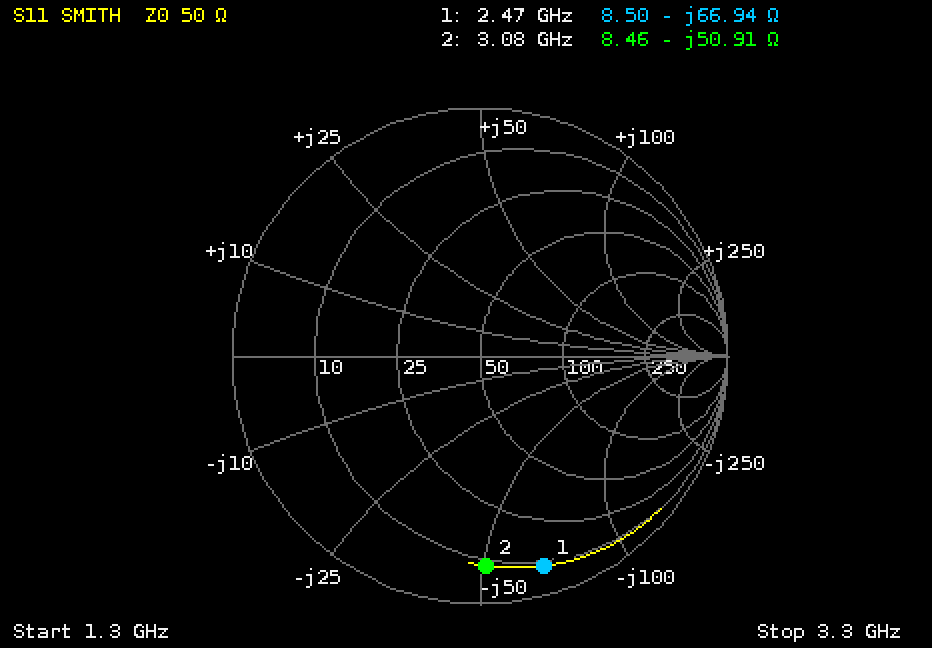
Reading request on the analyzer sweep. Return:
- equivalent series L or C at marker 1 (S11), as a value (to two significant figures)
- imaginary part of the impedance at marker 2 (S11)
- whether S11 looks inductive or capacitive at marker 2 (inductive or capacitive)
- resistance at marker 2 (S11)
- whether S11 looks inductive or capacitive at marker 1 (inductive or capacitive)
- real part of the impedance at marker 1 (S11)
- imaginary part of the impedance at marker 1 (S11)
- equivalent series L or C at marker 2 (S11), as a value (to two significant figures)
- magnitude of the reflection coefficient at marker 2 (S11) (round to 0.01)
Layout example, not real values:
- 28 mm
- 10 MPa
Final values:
- 960 fF
- -50.91 Ω
- capacitive
- 8.46 Ω
- capacitive
- 8.50 Ω
- -66.94 Ω
- 1.0 pF
- 0.85
